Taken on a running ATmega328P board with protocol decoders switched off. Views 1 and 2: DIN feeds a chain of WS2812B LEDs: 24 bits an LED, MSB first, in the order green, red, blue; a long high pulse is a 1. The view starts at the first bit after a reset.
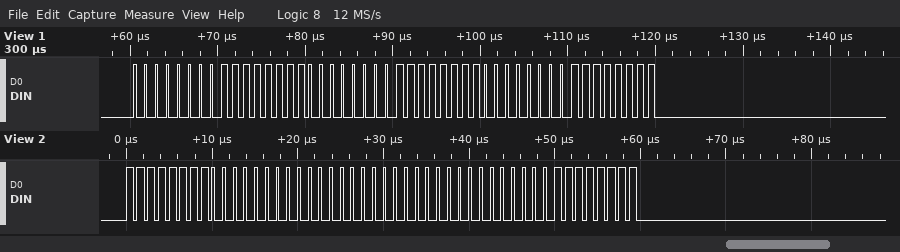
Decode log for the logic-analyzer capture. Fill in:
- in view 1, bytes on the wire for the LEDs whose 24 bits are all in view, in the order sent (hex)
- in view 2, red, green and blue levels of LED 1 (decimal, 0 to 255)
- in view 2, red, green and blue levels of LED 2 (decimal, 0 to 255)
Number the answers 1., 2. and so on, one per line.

1. 00 FF 00 FF 00 FF
2. 0, 255, 0
3. 0, 0, 255
